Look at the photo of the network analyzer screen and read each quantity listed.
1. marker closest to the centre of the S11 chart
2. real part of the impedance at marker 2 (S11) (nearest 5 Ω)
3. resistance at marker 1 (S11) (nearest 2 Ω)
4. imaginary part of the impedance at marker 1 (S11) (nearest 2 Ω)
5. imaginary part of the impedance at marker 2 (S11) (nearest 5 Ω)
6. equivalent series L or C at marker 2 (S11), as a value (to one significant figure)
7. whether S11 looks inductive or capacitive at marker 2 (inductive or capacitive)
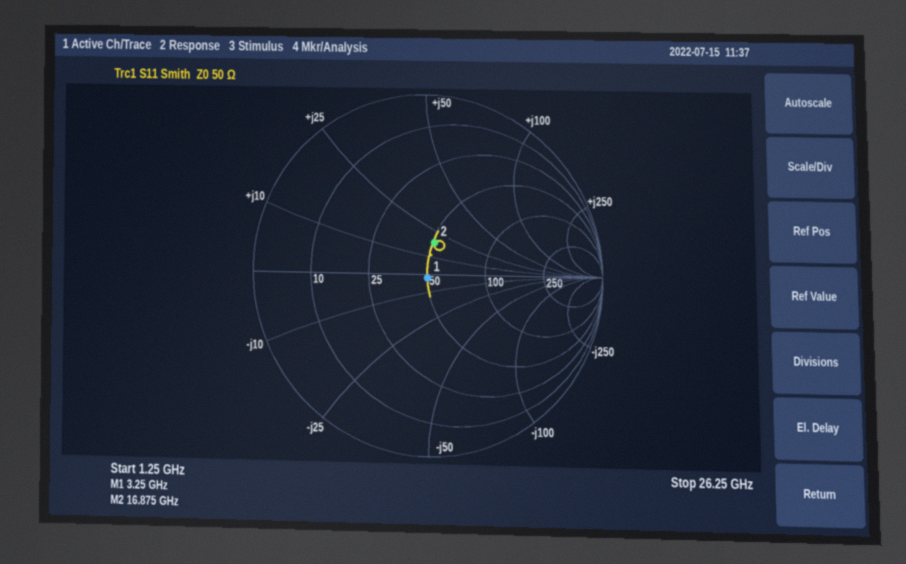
marker 1
50 Ω
50 Ω
-2 Ω
+20 Ω
200 pH
inductive
